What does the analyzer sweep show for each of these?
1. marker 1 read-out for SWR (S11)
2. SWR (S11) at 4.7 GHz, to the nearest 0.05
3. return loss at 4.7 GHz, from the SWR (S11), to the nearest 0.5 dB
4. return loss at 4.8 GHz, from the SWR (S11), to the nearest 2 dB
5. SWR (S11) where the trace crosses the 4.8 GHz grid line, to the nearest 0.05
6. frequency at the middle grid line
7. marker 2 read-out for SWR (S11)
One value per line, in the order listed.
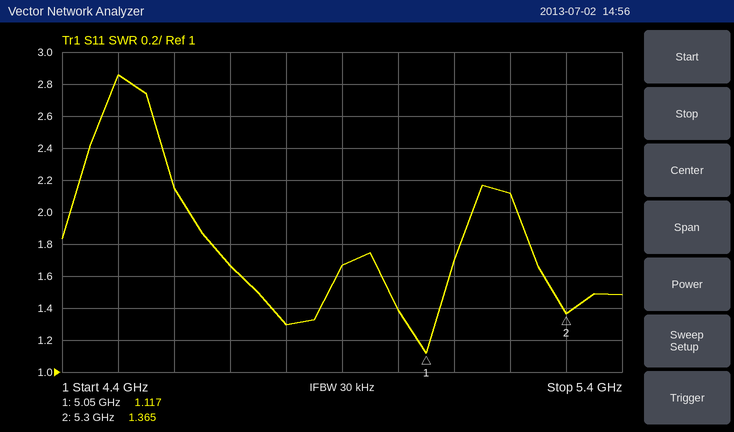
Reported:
1.117
1.65
12.0 dB
18 dB
1.30
4.9 GHz
1.365
